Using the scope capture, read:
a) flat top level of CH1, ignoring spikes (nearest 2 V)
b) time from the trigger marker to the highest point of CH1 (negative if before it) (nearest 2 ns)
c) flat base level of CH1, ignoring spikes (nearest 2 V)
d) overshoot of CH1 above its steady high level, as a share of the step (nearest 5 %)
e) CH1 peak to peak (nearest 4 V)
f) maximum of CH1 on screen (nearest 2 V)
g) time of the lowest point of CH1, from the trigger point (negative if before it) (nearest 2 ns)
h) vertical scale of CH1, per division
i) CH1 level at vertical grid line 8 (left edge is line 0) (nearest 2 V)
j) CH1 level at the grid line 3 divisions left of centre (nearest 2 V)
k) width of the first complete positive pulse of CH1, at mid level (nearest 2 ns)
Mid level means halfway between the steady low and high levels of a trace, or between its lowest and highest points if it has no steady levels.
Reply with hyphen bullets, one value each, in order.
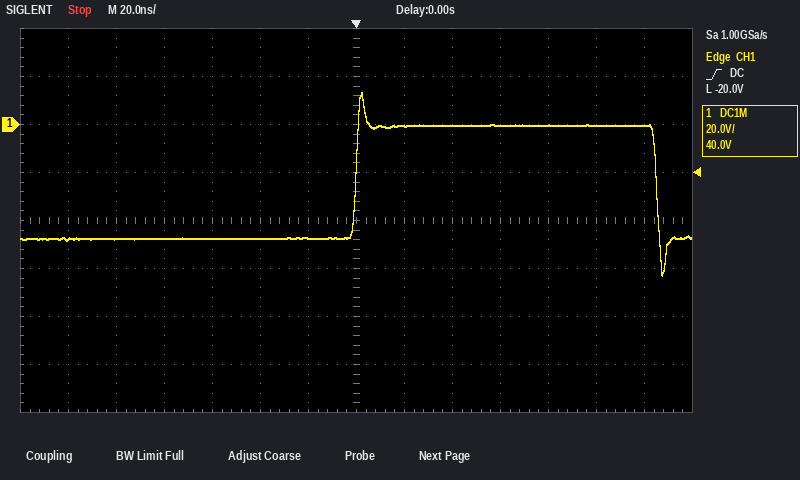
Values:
- 0 V
- +2 ns
- -48 V
- 30 %
- 76 V
- 14 V
- +128 ns
- 20 V
- 0 V
- -48 V
- 126 ns
